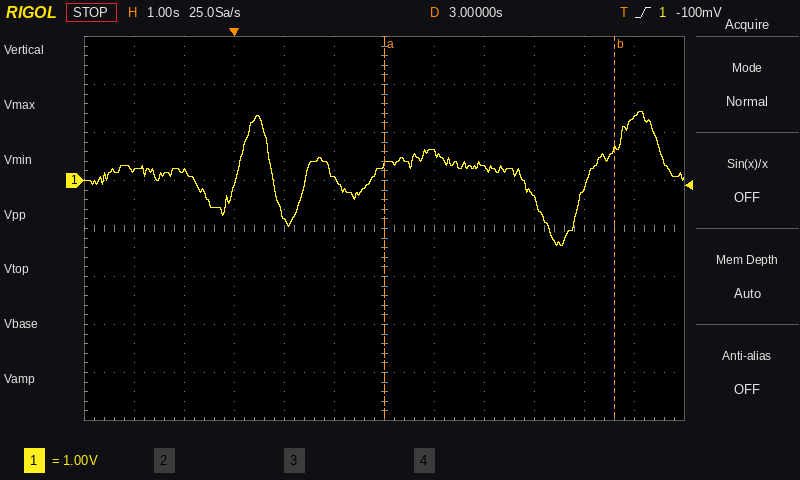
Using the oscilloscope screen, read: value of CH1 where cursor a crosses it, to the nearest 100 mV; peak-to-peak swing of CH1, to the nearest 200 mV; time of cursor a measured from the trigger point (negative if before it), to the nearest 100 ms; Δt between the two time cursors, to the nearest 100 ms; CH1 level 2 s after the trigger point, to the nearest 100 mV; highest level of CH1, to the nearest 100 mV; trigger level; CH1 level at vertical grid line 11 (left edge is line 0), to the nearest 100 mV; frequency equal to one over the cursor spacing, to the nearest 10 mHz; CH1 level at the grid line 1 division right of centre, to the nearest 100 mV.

300 mV
2.8 V
+3.0 s
4.6 s
0.0 V
1.4 V
-100 mV
1.3 V
220 mHz
600 mV
